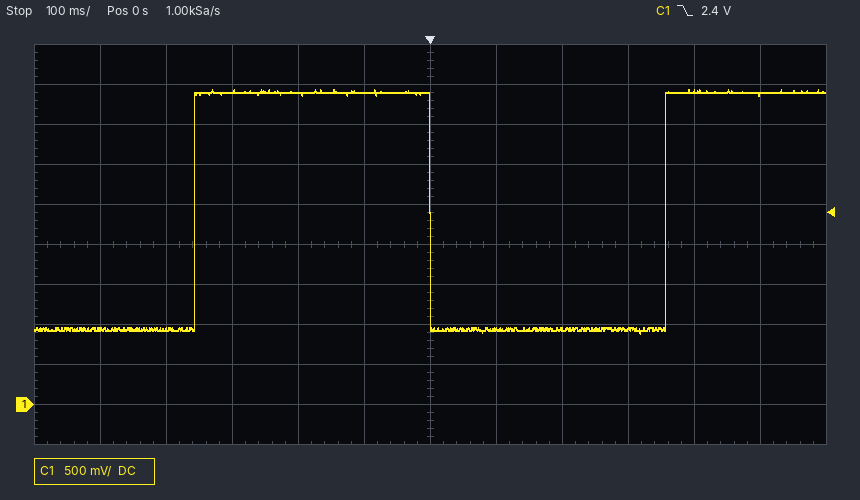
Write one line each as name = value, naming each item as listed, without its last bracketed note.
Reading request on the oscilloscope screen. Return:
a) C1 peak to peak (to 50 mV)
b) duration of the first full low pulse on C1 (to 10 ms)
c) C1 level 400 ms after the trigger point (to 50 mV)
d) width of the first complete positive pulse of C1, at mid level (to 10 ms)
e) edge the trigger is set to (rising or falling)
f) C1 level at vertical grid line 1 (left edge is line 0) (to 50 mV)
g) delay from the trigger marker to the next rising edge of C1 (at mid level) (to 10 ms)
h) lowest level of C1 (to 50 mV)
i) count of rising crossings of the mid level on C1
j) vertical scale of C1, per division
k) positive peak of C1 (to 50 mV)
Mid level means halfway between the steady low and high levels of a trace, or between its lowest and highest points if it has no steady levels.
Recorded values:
C1 peak to peak = 3.05 V
duration of the first full low pulse on C1 = 360 ms
C1 level 400 ms after the trigger point = 3.90 V
width of the first complete positive pulse of C1, at mid level = 360 ms
edge the trigger is set to = falling
C1 level at vertical grid line 1 (left edge is line 0) = 950 mV
delay from the trigger marker to the next rising edge of C1 (at mid level) = 360 ms
lowest level of C1 = 900 mV
count of rising crossings of the mid level on C1 = 2
vertical scale of C1, per division = 500 mV
positive peak of C1 = 3.95 V
